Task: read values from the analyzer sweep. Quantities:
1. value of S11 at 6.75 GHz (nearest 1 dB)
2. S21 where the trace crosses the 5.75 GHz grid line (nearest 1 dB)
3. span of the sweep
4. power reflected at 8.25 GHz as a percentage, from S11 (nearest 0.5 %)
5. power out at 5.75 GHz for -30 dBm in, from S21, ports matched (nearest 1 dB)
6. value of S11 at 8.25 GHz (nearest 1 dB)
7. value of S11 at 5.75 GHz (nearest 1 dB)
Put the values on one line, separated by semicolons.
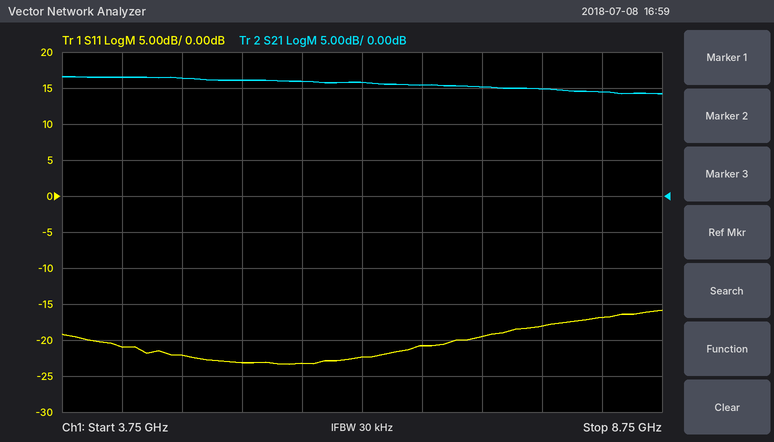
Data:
-21 dB; 16 dB; 5 GHz; 2.0 %; -14 dBm; -17 dB; -23 dB
